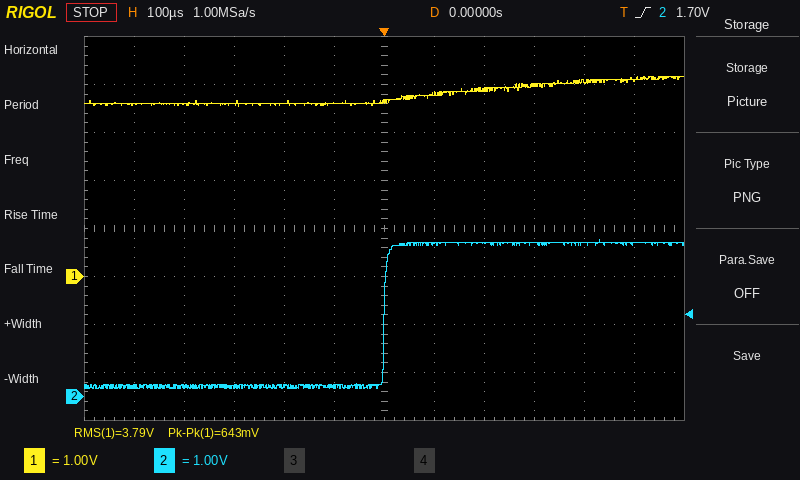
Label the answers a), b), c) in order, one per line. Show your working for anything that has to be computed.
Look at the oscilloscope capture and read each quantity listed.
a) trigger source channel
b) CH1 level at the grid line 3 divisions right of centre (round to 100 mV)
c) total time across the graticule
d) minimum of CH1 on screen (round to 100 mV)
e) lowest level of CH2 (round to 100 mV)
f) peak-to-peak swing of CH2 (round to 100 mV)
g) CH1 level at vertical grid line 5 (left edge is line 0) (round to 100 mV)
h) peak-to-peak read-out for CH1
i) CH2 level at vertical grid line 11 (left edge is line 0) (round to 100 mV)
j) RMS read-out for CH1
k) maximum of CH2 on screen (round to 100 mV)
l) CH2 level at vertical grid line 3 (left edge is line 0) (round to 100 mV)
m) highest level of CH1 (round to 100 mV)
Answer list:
a) CH2
b) 4.0 V
c) 1.2 ms
d) 3.5 V
e) 200 mV
f) 3.3 V − (200 mV) = 3.1 V
g) 3.6 V
h) 643 mV
i) 3.2 V
j) 3.79 V
k) 3.3 V
l) 200 mV
m) 4.2 V
